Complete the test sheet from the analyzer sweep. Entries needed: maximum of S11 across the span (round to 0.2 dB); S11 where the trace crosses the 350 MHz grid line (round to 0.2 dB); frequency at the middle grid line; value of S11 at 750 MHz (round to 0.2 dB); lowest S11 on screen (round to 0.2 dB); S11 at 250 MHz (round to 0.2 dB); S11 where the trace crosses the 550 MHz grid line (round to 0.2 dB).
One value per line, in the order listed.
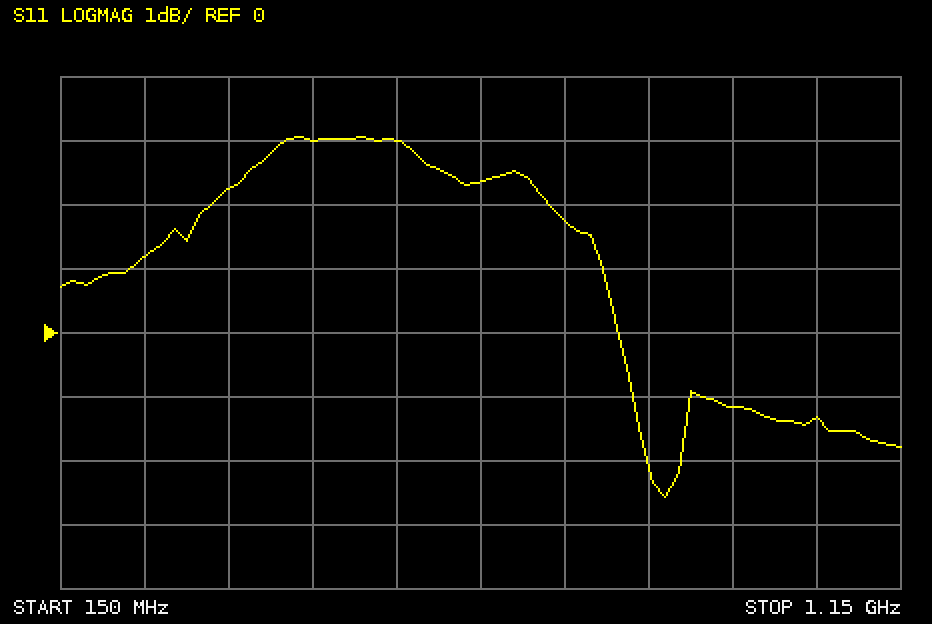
3.0 dB
2.2 dB
650 MHz
1.8 dB
-2.6 dB
1.2 dB
3.0 dB
